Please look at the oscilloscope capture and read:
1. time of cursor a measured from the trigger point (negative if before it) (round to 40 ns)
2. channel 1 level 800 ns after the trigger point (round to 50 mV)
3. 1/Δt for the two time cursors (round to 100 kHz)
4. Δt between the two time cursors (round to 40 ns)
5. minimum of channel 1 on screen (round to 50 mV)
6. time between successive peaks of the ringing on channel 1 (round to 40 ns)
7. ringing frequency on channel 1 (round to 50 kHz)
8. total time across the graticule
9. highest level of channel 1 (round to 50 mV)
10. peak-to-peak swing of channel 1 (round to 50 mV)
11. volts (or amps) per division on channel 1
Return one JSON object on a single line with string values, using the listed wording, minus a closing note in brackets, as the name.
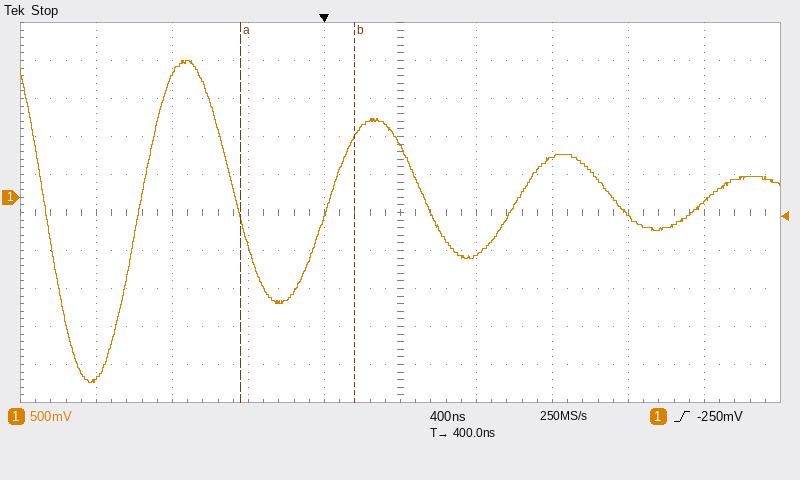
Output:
{"time of cursor a measured from the trigger point (negative if before it)": "-440 ns", "channel 1 level 800 ns after the trigger point": "-750 mV", "1/Δt for the two time cursors": "1.7 MHz", "Δt between the two time cursors": "600 ns", "minimum of channel 1 on screen": "-2.45 V", "time between successive peaks of the ringing on channel 1": "1.00 µs", "ringing frequency on channel 1": "1.00 MHz", "total time across the graticule": "4 µs", "highest level of channel 1": "1.80 V", "peak-to-peak swing of channel 1": "4.25 V", "volts (or amps) per division on channel 1": "500 mV"}
